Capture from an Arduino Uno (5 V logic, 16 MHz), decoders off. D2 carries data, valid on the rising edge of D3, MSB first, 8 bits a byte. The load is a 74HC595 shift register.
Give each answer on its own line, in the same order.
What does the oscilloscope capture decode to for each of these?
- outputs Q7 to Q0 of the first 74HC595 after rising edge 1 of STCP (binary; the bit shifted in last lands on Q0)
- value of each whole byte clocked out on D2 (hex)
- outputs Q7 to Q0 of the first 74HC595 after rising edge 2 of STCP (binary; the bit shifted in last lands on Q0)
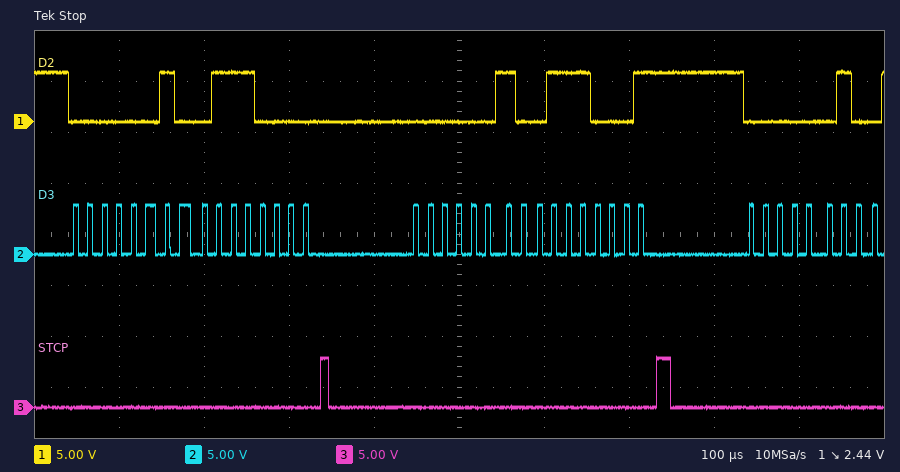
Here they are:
01110000
02 70 02 71 02
01110001
